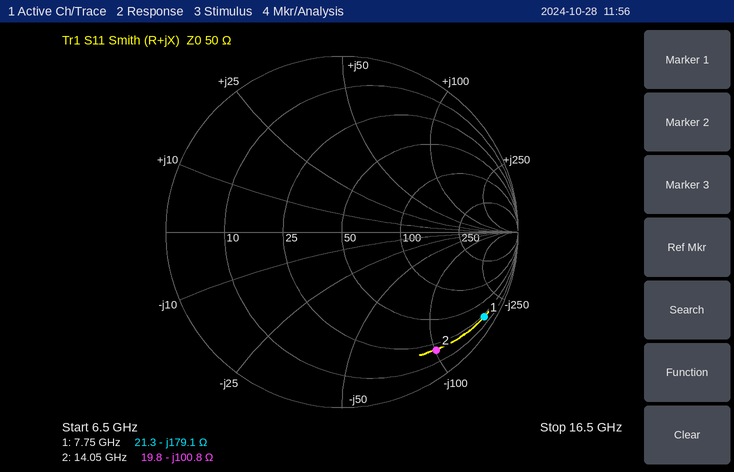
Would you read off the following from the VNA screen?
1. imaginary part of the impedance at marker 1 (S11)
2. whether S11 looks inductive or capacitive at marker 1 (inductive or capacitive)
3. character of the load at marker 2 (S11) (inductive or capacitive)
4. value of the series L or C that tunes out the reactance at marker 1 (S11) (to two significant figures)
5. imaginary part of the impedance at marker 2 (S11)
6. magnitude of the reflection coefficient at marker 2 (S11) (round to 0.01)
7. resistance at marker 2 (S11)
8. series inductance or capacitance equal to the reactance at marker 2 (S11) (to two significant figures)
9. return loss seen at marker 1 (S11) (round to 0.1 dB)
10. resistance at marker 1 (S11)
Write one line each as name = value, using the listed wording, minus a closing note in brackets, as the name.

imaginary part of the impedance at marker 1 = -179.1 Ω
whether S11 looks inductive or capacitive at marker 1 = capacitive
character of the load at marker 2 (S11) = capacitive
value of the series L or C that tunes out the reactance at marker 1 (S11) = 3.7 nH
imaginary part of the impedance at marker 2 = -100.8 Ω
magnitude of the reflection coefficient at marker 2 (S11) = 0.86
resistance at marker 2 = 19.8 Ω
series inductance or capacitance equal to the reactance at marker 2 (S11) = 110 fF
return loss seen at marker 1 (S11) = 0.5 dB
resistance at marker 1 = 21.3 Ω
